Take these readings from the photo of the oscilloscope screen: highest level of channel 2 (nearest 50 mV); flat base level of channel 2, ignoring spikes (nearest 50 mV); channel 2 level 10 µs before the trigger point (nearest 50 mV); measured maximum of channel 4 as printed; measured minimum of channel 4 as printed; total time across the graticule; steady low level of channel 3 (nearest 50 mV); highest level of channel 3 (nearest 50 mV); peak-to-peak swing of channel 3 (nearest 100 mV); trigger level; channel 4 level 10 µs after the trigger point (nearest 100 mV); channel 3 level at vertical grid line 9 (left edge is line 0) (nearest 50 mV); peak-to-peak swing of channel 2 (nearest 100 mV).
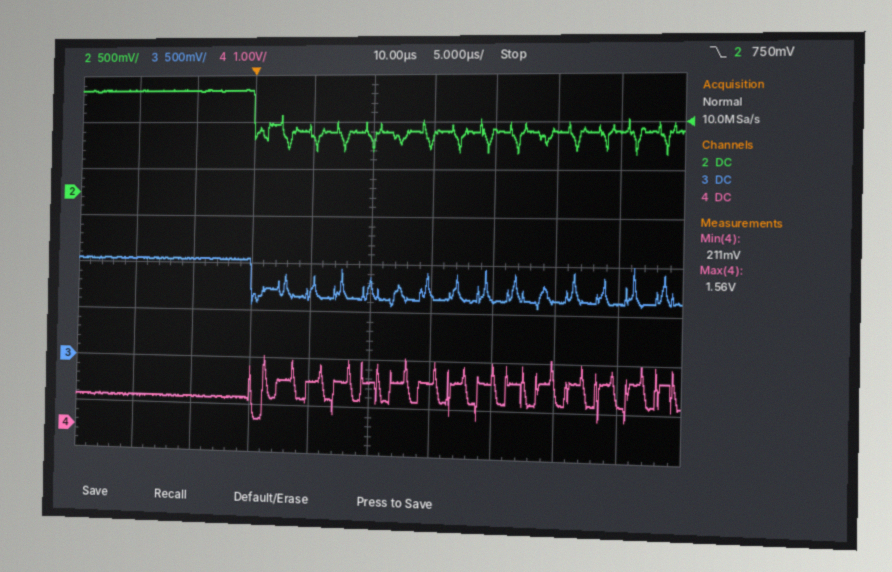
1.10 V
650 mV
1.10 V
1.56 V
211 mV
50 µs
650 mV
1.05 V
500 mV
750 mV
1.0 V
650 mV
700 mV
